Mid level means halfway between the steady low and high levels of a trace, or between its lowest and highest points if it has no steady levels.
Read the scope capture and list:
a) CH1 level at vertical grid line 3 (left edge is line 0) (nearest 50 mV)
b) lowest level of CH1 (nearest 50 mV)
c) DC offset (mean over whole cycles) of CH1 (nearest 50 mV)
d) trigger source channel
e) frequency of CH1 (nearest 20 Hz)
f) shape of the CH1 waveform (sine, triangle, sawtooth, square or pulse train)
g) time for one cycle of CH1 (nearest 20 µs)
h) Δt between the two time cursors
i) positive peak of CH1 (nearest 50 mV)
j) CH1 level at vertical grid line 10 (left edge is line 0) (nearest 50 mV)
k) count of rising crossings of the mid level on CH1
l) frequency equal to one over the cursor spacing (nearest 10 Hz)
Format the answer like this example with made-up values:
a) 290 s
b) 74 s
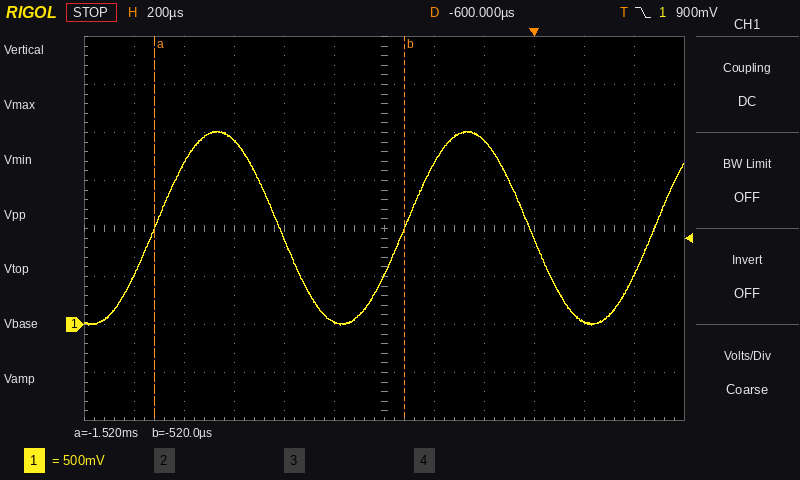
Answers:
a) 1.90 V
b) 0 mV
c) 1.00 V
d) CH1
e) 1.00 kHz
f) sine
g) 1.00 ms
h) 1.00 ms
i) 2.00 V
j) 50 mV
k) 3
l) 1.00 kHz
